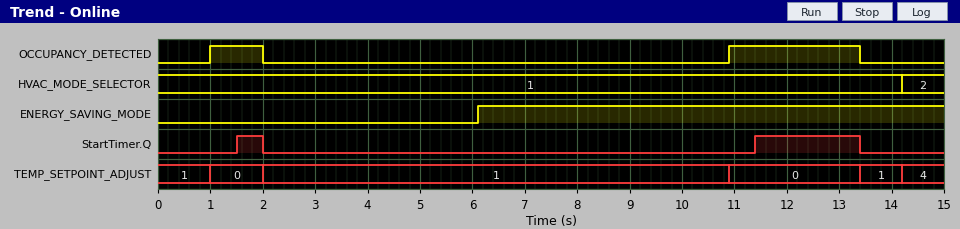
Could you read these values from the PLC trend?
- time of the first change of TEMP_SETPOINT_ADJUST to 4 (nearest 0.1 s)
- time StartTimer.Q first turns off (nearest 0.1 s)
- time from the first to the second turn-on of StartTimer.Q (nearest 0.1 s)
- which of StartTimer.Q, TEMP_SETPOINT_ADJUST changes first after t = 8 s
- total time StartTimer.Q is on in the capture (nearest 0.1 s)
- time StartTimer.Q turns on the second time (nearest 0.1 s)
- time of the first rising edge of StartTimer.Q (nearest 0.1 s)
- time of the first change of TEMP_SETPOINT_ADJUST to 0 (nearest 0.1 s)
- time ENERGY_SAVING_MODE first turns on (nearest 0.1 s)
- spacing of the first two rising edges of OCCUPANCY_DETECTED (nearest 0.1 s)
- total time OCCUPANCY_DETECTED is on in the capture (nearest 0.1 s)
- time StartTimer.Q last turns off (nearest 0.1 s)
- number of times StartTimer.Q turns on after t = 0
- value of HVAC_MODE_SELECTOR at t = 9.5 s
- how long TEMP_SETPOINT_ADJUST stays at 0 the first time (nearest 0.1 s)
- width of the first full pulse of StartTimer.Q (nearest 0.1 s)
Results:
14.2 s
2.0 s
9.9 s
TEMP_SETPOINT_ADJUST
2.5 s
11.4 s
1.5 s
1.0 s
6.1 s
9.9 s
3.5 s
13.4 s
2
1
1.0 s
0.5 s
